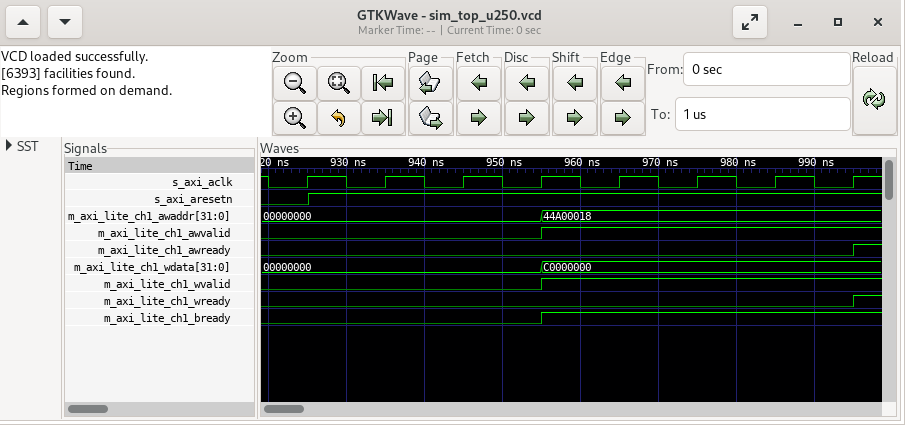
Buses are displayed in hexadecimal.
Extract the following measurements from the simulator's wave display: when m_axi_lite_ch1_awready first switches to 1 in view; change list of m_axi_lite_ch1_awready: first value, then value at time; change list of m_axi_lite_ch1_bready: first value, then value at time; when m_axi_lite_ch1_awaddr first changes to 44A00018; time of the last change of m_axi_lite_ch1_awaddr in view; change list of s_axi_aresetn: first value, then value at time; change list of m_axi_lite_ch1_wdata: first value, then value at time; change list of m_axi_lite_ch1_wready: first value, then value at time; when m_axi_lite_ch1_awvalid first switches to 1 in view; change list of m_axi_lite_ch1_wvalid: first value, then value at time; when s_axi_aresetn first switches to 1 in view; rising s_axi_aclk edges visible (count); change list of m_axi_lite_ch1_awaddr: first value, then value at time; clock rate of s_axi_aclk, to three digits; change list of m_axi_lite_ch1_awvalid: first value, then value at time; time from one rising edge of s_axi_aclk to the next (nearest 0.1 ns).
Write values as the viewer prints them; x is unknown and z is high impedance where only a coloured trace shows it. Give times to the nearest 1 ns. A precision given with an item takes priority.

995 ns
0, 1 at 995 ns
0, 1 at 955 ns
955 ns
955 ns
0, 1 at 925 ns
00000000, C0000000 at 955 ns
0, 1 at 995 ns
955 ns
0, 1 at 955 ns
925 ns
8
00000000, 44A00018 at 955 ns
100 MHz
0, 1 at 955 ns
10 ns
